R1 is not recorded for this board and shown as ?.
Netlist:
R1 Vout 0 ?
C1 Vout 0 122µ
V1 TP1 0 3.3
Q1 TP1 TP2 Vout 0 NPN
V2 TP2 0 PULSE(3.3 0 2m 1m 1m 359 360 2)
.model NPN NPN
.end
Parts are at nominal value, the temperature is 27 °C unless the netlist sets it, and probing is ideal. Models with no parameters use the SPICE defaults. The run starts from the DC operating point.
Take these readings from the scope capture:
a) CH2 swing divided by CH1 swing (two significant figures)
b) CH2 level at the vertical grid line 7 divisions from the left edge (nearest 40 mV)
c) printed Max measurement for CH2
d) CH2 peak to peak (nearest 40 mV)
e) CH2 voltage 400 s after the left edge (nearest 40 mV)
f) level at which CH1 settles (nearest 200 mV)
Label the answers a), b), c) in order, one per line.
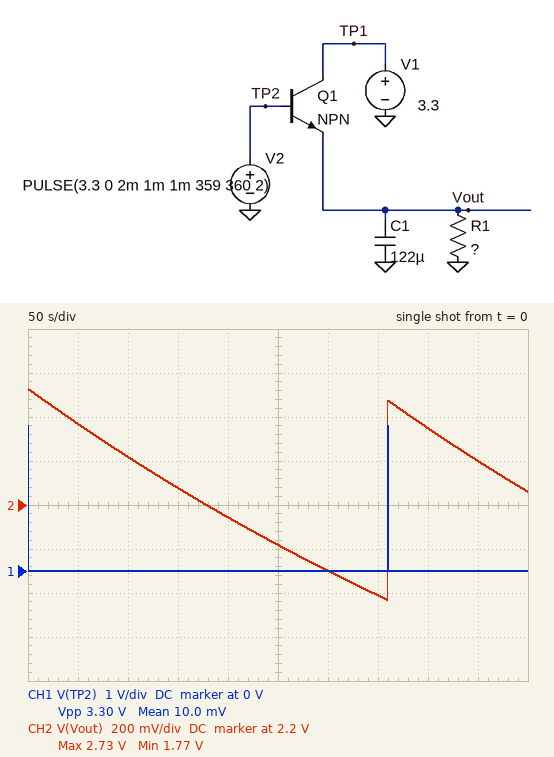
a) 0.29
b) 1.80 V
c) 2.73 V
d) 960 mV
e) 2.56 V
f) 0 V
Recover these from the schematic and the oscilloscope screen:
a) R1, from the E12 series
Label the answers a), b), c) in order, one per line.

a) 6.8 MΩ
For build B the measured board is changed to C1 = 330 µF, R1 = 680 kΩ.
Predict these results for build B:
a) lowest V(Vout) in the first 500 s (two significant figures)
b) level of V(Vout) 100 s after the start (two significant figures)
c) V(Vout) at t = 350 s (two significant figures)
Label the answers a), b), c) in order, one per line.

a) 540 mV
b) 1.7 V
c) 560 mV
